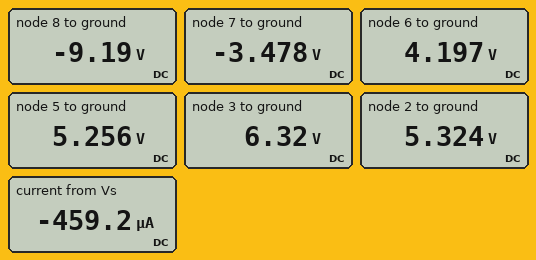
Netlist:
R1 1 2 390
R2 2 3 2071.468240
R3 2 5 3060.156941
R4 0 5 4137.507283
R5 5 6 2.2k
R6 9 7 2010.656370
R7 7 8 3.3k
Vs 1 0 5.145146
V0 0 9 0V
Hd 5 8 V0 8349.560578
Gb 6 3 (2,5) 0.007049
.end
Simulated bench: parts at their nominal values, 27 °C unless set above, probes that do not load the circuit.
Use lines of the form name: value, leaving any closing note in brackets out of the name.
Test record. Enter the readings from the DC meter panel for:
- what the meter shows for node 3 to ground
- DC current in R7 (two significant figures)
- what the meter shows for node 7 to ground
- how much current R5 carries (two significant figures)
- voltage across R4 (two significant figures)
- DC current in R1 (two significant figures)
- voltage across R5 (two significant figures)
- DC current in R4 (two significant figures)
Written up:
what the meter shows for node 3 to ground: 6.32 V
DC current in R7: 1.7 mA
what the meter shows for node 7 to ground: -3.478 V
how much current R5 carries: 480 µA
voltage across R4: 5.3 V
DC current in R1: 460 µA
voltage across R5: 1.1 V
DC current in R4: 1.3 mA
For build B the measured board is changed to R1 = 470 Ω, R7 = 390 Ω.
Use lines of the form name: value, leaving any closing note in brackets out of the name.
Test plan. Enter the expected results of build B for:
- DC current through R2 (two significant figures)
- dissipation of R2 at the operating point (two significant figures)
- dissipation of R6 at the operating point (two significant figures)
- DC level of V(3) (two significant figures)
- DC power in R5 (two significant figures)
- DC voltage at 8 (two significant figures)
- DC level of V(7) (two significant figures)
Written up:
DC current through R2: 390 µA
dissipation of R2 at the operating point: 310 µW
dissipation of R6 at the operating point: 1.4 mW
DC level of V(3): 4.2 V
DC power in R5: 330 µW
DC voltage at 8: -2.0 V
DC level of V(7): -1.7 V
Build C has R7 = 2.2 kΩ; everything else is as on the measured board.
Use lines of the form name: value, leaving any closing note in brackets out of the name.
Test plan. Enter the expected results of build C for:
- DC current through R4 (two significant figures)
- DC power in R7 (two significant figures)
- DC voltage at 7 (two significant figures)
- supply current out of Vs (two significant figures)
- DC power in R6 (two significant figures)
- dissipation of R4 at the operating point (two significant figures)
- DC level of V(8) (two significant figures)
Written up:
DC current through R4: 1.2 mA
DC power in R7: 3.4 mW
DC voltage at 7: -2.5 V
supply current out of Vs: 420 nA
DC power in R6: 3.1 mW
dissipation of R4 at the operating point: 6.4 mW
DC level of V(8): -5.2 V
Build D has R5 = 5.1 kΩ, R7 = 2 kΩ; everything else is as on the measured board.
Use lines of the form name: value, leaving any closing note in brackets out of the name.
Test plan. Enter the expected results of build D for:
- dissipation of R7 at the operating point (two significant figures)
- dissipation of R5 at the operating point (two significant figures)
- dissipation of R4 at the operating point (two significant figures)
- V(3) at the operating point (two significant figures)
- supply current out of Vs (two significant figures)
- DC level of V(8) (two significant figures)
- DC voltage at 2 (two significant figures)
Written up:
dissipation of R7 at the operating point: 2.8 mW
dissipation of R5 at the operating point: 19 µW
dissipation of R4 at the operating point: 6.4 mW
V(3) at the operating point: 5.0 V
supply current out of Vs: 58 µA
DC level of V(8): -4.7 V
DC voltage at 2: 5.1 V
